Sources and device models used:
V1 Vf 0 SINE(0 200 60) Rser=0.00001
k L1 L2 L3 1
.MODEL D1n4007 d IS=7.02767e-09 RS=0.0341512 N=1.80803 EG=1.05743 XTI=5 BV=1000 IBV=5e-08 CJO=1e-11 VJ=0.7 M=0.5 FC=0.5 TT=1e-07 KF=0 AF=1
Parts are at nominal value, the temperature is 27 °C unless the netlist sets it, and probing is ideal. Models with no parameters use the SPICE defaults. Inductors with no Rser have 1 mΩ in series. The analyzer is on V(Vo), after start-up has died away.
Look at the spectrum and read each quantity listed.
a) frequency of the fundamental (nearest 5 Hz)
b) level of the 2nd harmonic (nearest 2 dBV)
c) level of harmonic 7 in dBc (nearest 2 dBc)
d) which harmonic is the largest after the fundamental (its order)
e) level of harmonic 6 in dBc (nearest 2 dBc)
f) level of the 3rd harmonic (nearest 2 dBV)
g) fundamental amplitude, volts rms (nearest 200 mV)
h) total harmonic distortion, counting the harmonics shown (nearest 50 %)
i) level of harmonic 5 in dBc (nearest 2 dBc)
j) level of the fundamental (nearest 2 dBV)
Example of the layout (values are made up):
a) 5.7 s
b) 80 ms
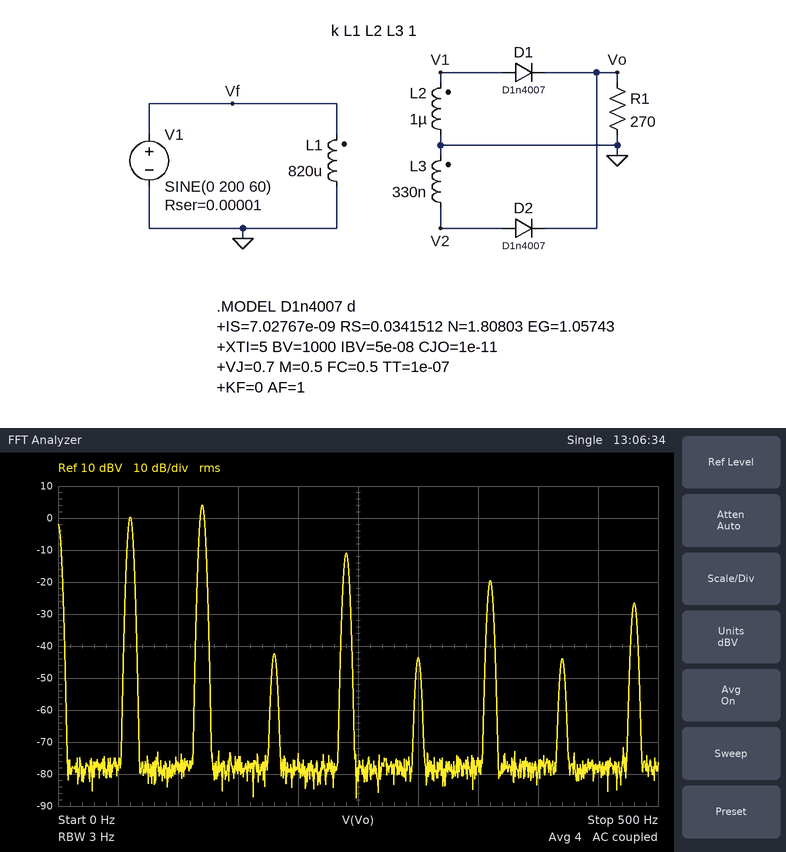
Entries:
a) 60 Hz
b) 4 dBV
c) -44 dBc
d) 2
e) -20 dBc
f) -42 dBV
g) 1.0 V
h) 150 %
i) -44 dBc
j) 0 dBV
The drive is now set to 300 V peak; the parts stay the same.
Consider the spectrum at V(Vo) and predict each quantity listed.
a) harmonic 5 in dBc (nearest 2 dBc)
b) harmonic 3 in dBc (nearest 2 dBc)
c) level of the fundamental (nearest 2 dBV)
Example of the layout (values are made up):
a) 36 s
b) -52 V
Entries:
a) -50 dBc
b) -48 dBc
c) 4 dBV
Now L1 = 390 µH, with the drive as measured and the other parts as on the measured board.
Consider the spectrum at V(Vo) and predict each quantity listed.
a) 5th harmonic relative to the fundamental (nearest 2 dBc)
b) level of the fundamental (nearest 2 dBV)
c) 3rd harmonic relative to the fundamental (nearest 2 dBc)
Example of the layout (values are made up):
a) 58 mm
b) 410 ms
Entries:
a) -50 dBc
b) 4 dBV
c) -48 dBc
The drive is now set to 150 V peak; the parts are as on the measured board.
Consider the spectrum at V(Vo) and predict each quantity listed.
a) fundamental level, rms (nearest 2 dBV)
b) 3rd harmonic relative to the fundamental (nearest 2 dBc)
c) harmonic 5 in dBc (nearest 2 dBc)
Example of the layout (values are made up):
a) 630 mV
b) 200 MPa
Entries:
a) -2 dBV
b) -38 dBc
c) -40 dBc
